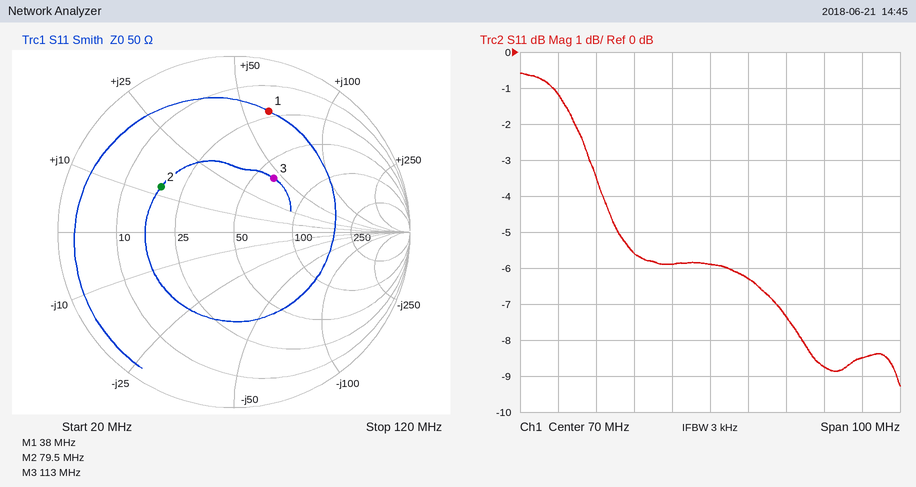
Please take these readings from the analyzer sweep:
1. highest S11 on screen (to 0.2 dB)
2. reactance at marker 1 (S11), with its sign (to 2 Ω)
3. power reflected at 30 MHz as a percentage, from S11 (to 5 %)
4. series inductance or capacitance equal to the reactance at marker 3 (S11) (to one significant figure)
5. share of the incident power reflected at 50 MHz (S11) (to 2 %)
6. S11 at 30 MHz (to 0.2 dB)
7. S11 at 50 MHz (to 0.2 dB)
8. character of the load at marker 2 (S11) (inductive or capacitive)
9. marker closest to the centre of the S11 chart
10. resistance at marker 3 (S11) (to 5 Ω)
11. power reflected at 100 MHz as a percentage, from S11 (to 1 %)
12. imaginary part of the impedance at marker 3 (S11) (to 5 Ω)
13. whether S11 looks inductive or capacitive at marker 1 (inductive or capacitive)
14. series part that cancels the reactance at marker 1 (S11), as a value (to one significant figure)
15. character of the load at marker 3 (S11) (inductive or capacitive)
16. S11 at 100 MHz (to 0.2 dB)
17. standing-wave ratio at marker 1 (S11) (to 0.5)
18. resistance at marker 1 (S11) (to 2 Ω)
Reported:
-0.6 dB
+62 Ω
75 %
60 nH
28 %
-1.2 dB
-5.6 dB
inductive
marker 3
60 Ω
13 %
+45 Ω
inductive
70 pF
inductive
-8.8 dB
6.0
22 Ω
